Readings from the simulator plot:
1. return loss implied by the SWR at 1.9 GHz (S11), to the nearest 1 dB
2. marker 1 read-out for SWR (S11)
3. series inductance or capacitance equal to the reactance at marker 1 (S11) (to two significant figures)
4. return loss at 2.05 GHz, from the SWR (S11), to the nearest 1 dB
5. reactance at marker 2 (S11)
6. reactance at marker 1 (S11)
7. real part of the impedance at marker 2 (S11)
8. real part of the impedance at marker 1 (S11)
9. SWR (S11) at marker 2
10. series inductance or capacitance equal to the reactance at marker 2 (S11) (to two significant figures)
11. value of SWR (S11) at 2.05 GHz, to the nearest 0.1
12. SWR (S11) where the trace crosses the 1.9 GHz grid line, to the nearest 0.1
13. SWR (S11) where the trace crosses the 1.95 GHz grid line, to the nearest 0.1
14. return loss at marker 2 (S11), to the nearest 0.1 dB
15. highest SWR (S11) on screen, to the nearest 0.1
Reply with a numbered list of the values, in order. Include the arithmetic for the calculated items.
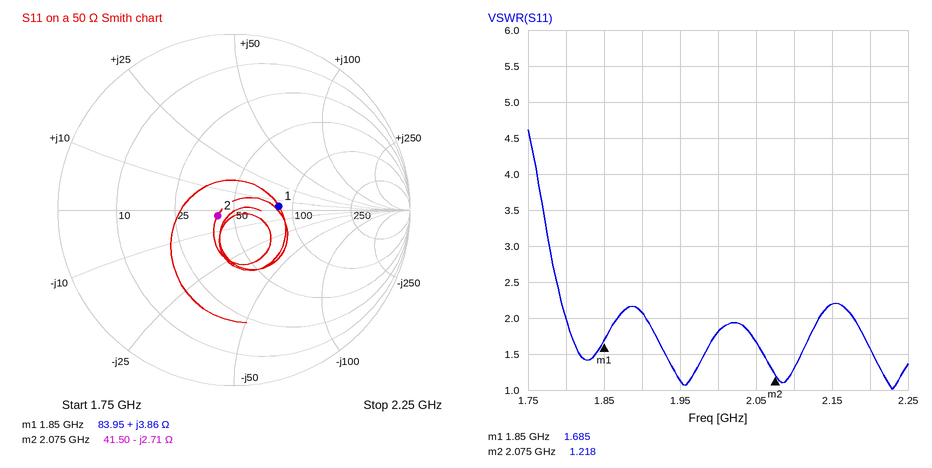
1. −20 log10((2.1 − 1)/(2.1 + 1)) ≈ 9 dB
2. 1.685
3. L = 3.86 Ω/(2π × 1.85 GHz) ≈ 332 pH, so 330 pH to two significant figures
4. −20 log10((1.7 − 1)/(1.7 + 1)) ≈ 12 dB
5. -2.71 Ω
6. +3.86 Ω
7. 41.50 Ω
8. 83.95 Ω
9. 1.218
10. C = 1/(2π × 2.075 GHz × 2.71 Ω) ≈ 28 pF
11. 1.7
12. 2.1
13. 1.1
14. 20.2 dB
15. 4.6
